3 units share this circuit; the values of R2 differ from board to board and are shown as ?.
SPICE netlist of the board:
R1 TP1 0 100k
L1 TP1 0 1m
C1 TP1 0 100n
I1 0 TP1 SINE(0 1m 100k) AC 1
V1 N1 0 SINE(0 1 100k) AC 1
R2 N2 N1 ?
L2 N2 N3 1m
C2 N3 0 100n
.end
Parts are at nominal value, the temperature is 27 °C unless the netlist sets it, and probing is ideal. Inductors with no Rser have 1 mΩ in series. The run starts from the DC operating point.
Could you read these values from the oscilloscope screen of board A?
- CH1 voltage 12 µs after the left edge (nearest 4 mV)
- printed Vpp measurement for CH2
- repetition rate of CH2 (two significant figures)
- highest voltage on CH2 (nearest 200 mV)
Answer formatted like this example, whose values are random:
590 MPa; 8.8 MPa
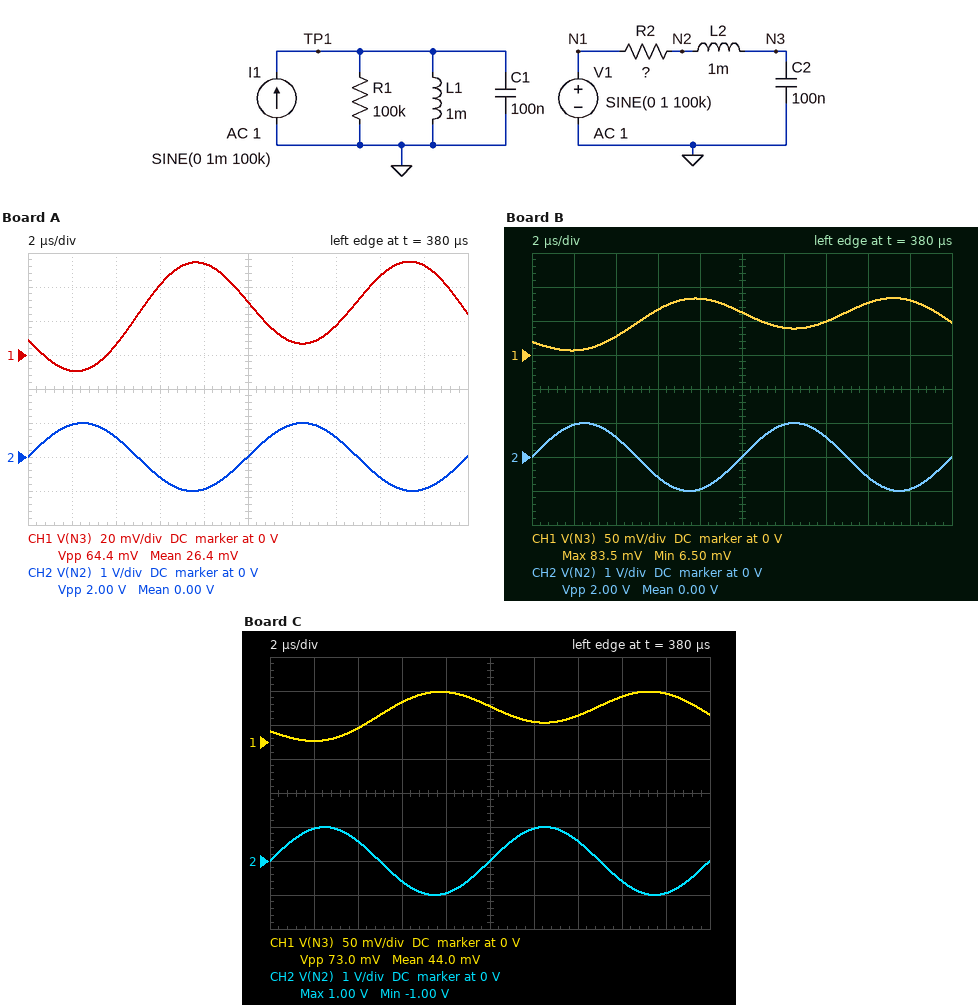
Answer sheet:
8 mV; 2.00 V; 100 kHz; 1.0 V
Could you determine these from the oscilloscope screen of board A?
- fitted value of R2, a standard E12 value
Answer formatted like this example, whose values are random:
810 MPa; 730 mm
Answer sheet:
8.2 Ω
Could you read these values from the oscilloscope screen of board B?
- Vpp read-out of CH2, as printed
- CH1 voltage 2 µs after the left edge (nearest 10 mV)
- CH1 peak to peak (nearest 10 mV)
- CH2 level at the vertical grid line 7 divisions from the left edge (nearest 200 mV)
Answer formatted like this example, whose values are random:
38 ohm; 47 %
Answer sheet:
2.00 V; 10 mV; 80 mV; 600 mV
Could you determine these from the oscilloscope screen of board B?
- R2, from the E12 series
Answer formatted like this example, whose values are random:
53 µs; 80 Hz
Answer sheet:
4.7 Ω
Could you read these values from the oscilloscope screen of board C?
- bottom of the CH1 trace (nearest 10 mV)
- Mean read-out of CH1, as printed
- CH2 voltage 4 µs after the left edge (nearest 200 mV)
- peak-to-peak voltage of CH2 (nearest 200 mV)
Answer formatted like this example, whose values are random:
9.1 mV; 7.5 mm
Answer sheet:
0 V; 44.0 mV; 600 mV; 2.0 V
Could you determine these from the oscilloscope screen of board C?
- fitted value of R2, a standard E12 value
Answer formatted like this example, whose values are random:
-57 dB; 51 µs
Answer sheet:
5.6 Ω
